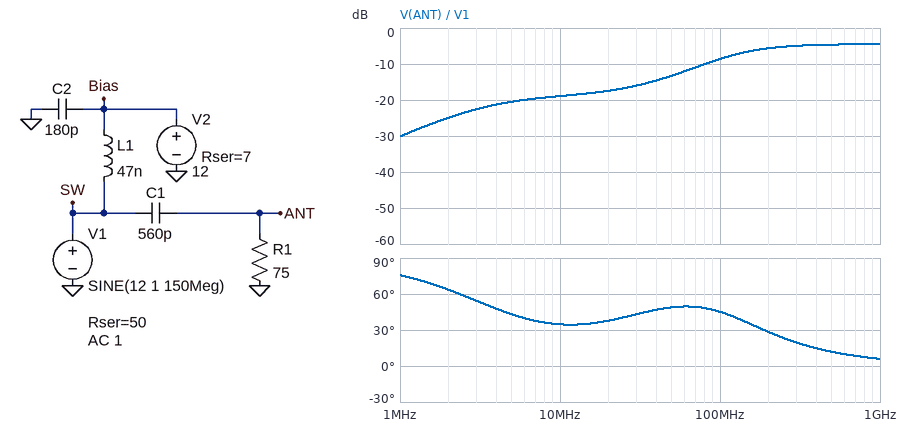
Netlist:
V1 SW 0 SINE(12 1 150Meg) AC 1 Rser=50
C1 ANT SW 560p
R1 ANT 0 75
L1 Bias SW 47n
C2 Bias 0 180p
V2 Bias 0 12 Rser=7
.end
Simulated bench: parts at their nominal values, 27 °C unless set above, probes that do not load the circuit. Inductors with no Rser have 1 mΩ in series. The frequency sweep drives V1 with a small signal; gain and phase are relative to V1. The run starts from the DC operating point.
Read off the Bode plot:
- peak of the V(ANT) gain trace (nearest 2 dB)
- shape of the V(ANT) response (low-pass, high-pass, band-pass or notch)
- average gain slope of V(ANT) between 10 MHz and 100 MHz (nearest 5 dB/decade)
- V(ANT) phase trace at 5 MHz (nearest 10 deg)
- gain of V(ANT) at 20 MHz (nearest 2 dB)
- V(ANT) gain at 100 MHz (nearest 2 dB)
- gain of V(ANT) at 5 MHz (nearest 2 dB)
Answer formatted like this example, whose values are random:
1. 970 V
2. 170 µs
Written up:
1. -4 dB
2. high-pass
3. 10 dB/decade
4. 40 deg
5. -18 dB
6. -8 dB
7. -20 dB
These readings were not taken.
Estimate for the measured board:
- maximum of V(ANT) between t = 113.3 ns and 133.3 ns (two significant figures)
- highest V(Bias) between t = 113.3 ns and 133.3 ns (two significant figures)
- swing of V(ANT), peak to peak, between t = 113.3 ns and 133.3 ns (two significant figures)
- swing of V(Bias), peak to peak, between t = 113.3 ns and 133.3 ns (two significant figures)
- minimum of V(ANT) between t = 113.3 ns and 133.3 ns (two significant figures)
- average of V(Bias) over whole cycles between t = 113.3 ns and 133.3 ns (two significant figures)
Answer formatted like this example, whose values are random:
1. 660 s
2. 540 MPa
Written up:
1. 470 mV
2. 12 V
3. 940 mV
4. 100 mV
5. -470 mV
6. 12 V
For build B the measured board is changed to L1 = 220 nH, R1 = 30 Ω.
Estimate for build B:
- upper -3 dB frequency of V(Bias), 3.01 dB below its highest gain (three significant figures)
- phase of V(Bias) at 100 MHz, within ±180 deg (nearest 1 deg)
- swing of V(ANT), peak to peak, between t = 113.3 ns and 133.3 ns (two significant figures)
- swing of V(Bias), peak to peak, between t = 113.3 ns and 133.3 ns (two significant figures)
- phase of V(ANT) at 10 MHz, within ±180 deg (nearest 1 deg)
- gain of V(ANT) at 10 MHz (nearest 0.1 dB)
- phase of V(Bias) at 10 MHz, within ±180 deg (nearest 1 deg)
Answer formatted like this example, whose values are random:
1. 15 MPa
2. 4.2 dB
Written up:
1. 18.6 MHz
2. -122 deg
3. 750 mV
4. 17 mV
5. 75 deg
6. -14.9 dB
7. -35 deg
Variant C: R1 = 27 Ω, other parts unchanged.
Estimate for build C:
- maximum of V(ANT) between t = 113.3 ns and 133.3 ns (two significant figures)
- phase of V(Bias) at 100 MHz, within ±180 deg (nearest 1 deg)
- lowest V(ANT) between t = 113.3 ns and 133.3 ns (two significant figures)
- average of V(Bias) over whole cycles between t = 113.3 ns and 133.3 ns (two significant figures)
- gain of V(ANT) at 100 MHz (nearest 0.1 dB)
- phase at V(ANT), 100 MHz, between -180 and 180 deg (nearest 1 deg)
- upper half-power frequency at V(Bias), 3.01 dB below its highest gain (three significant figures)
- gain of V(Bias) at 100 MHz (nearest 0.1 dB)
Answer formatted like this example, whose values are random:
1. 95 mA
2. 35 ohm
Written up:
1. 320 mV
2. -91 deg
3. -320 mV
4. 12 V
5. -11.1 dB
6. 34 deg
7. 55.5 MHz
8. -24.7 dB
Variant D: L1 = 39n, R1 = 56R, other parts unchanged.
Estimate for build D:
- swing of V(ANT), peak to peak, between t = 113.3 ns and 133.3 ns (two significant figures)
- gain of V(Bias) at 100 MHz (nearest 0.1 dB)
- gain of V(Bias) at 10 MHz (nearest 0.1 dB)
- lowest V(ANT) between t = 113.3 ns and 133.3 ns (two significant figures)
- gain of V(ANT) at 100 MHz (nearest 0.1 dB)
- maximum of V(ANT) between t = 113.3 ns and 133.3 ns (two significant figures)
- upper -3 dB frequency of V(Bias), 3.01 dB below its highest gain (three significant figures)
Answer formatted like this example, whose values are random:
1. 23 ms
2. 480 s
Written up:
1. 800 mV
2. -22.1 dB
3. -18.9 dB
4. -400 mV
5. -10.2 dB
6. 400 mV
7. 84.4 MHz
